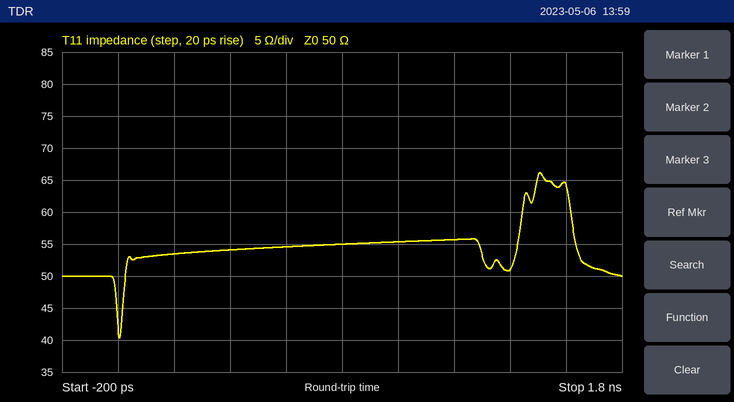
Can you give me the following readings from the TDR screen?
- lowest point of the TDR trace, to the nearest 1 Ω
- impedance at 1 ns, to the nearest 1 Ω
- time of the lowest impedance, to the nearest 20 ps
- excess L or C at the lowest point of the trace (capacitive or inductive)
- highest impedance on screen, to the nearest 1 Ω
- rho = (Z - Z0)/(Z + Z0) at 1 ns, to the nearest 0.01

40 Ω
55 Ω
0 ps
capacitive
66 Ω
+0.05
